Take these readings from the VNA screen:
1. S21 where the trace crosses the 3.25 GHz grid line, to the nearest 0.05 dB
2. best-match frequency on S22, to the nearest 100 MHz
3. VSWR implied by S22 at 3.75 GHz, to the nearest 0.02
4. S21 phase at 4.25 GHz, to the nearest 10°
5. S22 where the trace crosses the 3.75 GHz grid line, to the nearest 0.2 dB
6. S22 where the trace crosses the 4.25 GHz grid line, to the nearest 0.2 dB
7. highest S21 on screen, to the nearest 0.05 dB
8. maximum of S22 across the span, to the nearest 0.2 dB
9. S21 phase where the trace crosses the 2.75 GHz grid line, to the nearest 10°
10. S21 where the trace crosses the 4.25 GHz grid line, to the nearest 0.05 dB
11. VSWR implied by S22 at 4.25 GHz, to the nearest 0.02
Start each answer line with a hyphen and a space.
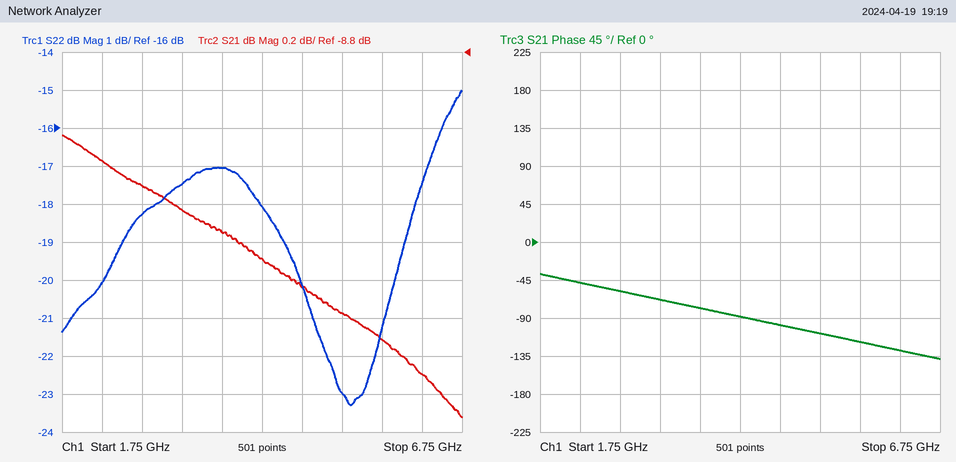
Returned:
- -9.65 dB
- 5.4 GHz
- 1.32
- -90°
- -17.0 dB
- -18.0 dB
- -9.25 dB
- -15.0 dB
- -60°
- -9.90 dB
- 1.28
